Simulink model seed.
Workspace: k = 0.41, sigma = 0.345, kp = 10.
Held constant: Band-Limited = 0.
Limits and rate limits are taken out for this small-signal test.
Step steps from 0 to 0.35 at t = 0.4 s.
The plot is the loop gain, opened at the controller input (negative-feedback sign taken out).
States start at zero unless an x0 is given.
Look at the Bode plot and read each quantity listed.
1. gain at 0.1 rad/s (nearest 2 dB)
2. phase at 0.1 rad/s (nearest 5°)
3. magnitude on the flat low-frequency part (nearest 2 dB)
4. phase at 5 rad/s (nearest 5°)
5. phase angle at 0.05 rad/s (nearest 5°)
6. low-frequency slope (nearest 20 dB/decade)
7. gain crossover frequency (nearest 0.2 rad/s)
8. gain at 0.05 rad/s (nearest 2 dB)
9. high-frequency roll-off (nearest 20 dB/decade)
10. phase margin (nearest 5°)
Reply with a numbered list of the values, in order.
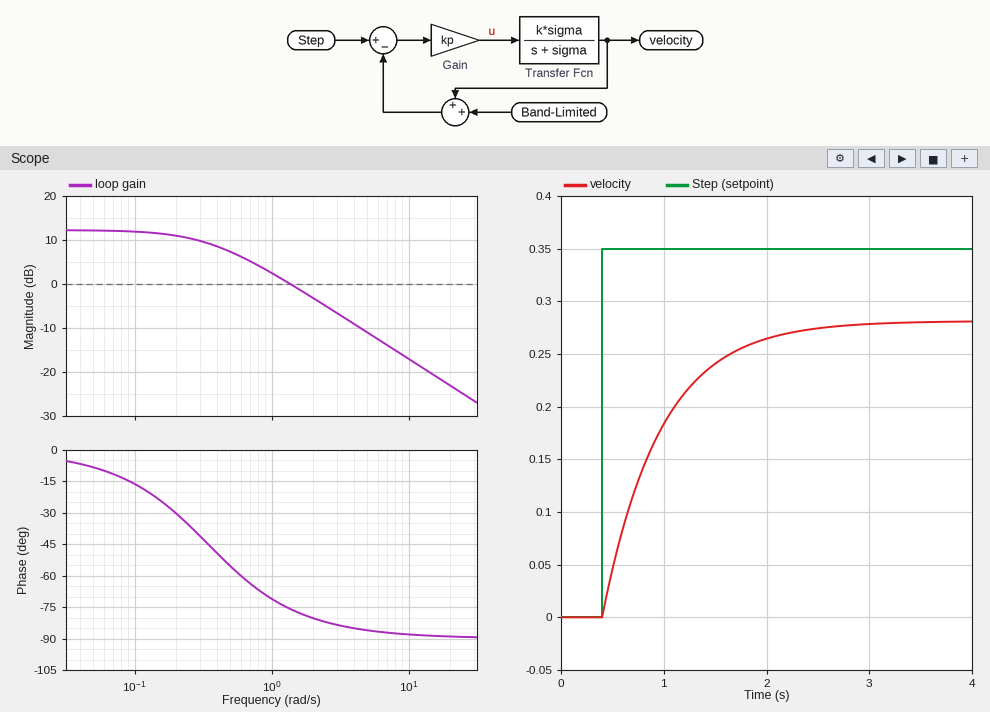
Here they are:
1. 12 dB
2. -15°
3. 12 dB
4. -85°
5. -10°
6. 0 dB/decade
7. 1.4 rad/s
8. 12 dB
9. -20 dB/decade
10. 105°
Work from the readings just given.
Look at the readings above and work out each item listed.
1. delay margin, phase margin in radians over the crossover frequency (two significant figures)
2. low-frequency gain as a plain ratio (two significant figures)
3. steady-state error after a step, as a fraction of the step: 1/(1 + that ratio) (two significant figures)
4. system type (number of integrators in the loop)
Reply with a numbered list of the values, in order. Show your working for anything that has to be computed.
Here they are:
1. 105 × π / 180 / 1.4 = 1.3 s
2. 10^(12 / 20) = 4.0
3. 1 / (1 + 4) = 0.20
4. 0
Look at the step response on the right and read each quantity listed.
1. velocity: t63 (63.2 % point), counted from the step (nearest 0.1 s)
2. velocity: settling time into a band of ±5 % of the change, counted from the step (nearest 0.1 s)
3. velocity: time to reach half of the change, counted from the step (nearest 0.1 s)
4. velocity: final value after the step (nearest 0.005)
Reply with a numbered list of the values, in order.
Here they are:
1. 0.6 s
2. 1.7 s
3. 0.4 s
4. 0.280
